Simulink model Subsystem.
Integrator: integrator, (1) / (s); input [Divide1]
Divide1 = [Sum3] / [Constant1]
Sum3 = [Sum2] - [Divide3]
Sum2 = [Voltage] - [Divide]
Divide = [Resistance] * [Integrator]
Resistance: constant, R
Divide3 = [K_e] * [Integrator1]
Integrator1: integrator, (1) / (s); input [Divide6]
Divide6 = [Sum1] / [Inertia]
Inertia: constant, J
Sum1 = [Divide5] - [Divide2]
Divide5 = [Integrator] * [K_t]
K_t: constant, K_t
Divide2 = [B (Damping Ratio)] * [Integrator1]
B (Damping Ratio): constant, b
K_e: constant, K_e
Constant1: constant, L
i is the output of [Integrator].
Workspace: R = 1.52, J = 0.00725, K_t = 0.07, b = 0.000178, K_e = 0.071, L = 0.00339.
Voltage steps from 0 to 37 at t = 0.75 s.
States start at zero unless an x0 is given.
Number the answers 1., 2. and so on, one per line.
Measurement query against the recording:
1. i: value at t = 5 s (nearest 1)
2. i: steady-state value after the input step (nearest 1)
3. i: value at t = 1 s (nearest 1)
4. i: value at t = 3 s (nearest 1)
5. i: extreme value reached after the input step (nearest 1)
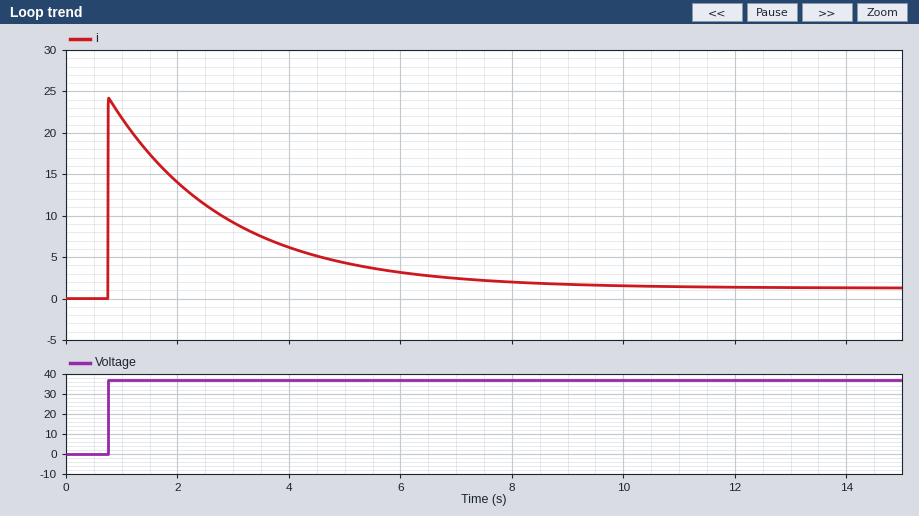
1. 4
2. 1
3. 22
4. 9
5. 24
